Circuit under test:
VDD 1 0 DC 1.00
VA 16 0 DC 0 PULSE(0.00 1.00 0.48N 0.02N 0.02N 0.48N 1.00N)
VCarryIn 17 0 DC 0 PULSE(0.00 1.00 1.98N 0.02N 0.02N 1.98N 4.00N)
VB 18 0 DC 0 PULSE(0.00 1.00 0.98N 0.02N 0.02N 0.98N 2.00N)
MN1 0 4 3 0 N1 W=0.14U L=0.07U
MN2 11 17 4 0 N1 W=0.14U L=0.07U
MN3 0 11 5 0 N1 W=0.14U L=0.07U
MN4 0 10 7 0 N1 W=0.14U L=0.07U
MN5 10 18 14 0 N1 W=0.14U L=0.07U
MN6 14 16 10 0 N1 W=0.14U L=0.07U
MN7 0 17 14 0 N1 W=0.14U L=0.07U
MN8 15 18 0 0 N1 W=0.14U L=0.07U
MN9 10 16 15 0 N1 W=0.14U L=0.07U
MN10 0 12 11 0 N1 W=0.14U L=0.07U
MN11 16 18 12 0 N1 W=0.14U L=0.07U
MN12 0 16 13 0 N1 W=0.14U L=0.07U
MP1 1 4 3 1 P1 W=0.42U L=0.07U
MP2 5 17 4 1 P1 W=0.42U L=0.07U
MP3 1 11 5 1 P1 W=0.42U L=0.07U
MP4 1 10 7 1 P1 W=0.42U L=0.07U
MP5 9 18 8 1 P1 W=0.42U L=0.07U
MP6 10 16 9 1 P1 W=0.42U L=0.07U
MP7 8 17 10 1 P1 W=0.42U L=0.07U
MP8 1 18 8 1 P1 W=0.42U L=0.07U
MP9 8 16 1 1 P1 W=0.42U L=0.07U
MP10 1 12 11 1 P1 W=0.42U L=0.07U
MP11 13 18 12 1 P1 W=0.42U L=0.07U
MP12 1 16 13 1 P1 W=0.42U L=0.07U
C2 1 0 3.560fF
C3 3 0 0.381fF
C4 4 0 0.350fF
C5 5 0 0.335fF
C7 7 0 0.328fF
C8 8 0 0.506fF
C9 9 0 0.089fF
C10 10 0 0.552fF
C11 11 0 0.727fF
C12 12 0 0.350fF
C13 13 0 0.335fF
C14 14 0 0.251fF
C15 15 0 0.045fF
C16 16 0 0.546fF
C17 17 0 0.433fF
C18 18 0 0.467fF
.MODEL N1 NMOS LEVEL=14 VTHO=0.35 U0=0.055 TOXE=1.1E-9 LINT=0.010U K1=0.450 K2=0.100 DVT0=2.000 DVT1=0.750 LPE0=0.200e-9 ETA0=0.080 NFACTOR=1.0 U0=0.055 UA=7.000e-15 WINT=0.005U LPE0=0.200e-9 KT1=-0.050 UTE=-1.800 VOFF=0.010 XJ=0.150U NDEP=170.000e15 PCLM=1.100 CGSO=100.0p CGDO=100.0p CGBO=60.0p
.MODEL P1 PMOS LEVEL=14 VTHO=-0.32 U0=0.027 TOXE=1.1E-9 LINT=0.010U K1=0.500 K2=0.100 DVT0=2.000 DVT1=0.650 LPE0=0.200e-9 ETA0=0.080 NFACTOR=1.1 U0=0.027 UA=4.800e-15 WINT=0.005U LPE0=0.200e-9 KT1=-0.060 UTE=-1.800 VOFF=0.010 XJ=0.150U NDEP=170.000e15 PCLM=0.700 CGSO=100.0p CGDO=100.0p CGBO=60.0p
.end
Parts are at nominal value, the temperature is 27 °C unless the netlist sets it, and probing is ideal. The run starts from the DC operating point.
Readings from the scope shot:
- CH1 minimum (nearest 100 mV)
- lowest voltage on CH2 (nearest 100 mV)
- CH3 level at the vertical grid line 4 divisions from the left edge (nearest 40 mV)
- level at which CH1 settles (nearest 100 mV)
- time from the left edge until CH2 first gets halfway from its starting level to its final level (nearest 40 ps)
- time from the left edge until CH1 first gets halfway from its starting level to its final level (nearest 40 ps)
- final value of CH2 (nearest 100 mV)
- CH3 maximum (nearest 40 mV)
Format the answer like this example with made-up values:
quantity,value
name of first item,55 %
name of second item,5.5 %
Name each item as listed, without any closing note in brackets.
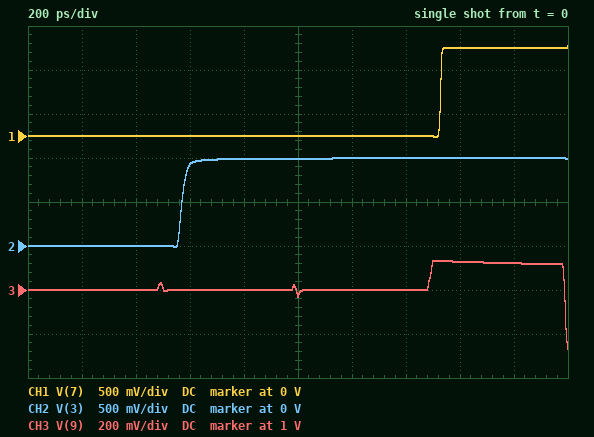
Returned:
quantity,value
CH1 minimum,0 V
lowest voltage on CH2,0 V
CH3 level at the vertical grid line 4 divisions from the left edge,1.00 V
level at which CH1 settles,1.0 V
time from the left edge until CH2 first gets halfway from its starting level to its final level,560 ps
time from the left edge until CH1 first gets halfway from its starting level to its final level,1.52 ns
final value of CH2,1.0 V
CH3 maximum,1.12 V
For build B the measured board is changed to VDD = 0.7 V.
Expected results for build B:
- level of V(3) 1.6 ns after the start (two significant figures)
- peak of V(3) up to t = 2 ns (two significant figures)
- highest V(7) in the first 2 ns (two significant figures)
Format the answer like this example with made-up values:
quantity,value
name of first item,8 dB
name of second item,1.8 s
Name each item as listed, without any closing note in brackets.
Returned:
quantity,value
level of V(3) 1.6 ns after the start,500 mV
peak of V(3) up to t = 2 ns,530 mV
highest V(7) in the first 2 ns,700 mV
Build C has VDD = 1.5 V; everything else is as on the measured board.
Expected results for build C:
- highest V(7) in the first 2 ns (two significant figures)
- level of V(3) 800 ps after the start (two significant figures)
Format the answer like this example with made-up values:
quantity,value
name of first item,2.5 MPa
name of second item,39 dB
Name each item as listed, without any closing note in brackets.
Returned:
quantity,value
highest V(7) in the first 2 ns,140 mV
level of V(3) 800 ps after the start,1.5 V
